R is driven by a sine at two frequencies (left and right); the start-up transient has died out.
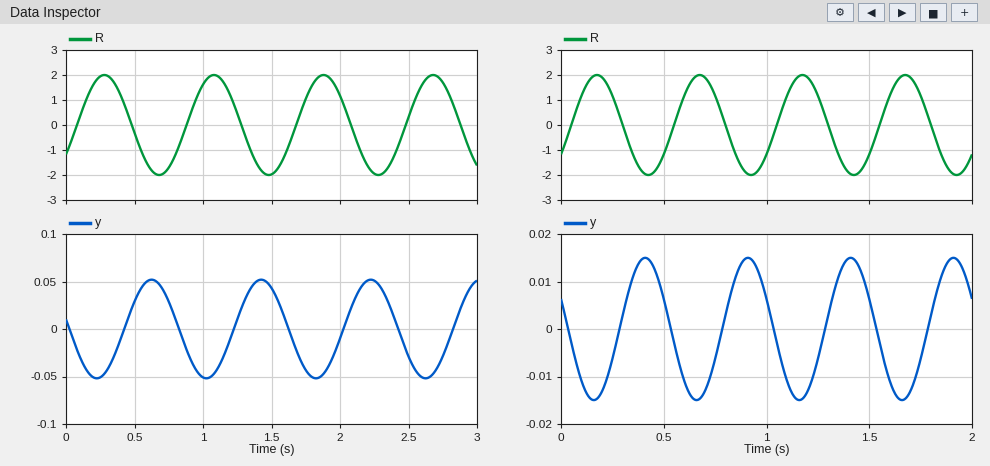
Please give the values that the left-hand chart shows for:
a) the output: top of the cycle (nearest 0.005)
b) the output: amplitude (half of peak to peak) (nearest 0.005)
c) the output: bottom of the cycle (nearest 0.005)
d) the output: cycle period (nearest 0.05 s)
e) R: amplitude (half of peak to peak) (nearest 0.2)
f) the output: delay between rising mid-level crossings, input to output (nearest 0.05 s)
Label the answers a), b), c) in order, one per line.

a) 0.050
b) 0.050
c) -0.050
d) 0.80 s
e) 2.0
f) 0.35 s
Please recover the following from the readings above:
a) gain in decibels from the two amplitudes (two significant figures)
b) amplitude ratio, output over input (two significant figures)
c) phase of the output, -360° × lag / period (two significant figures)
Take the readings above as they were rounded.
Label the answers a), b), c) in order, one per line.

a) -32 dB
b) 0.025
c) -160°
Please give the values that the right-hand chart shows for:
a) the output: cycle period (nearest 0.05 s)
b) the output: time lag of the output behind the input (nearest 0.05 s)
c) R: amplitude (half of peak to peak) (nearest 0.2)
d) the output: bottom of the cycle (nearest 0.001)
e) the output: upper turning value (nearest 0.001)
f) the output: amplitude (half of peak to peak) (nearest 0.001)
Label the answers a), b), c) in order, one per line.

a) 0.50 s
b) 0.25 s
c) 2.0
d) -0.015
e) 0.015
f) 0.015
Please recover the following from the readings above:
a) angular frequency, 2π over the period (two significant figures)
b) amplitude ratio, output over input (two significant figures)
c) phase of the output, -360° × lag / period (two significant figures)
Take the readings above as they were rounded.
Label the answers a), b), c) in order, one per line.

a) 13 rad/s
b) 0.0075
c) -180°
